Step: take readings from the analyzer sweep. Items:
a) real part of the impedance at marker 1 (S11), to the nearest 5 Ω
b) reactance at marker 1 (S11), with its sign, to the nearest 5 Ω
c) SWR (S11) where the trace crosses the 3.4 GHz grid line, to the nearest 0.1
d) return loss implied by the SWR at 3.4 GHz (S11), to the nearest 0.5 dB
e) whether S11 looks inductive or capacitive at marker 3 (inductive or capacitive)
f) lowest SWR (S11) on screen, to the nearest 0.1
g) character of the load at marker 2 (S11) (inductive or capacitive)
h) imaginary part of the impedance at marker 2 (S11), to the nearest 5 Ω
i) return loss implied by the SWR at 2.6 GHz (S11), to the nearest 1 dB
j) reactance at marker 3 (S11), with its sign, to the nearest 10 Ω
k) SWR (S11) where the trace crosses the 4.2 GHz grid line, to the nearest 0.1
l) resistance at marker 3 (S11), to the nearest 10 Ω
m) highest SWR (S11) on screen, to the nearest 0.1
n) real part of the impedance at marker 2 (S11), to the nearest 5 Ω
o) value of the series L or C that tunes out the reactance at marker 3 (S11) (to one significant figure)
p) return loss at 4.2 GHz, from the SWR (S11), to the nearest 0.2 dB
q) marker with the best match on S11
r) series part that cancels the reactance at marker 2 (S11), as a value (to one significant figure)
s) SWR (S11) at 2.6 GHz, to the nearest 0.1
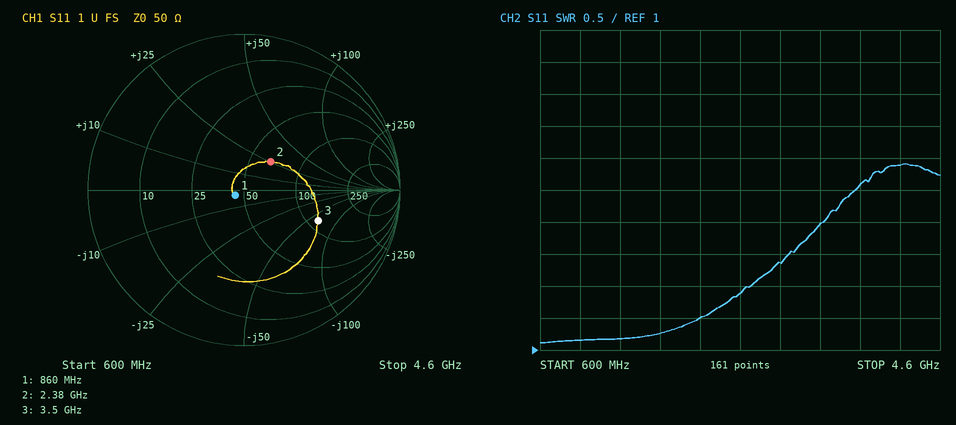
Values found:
45 Ω
-5 Ω
3.0
6.0 dB
capacitive
1.1
inductive
+25 Ω
10 dB
-60 Ω
3.9
120 Ω
3.9
65 Ω
3 nH
4.6 dB
marker 1
3 pF
1.9
